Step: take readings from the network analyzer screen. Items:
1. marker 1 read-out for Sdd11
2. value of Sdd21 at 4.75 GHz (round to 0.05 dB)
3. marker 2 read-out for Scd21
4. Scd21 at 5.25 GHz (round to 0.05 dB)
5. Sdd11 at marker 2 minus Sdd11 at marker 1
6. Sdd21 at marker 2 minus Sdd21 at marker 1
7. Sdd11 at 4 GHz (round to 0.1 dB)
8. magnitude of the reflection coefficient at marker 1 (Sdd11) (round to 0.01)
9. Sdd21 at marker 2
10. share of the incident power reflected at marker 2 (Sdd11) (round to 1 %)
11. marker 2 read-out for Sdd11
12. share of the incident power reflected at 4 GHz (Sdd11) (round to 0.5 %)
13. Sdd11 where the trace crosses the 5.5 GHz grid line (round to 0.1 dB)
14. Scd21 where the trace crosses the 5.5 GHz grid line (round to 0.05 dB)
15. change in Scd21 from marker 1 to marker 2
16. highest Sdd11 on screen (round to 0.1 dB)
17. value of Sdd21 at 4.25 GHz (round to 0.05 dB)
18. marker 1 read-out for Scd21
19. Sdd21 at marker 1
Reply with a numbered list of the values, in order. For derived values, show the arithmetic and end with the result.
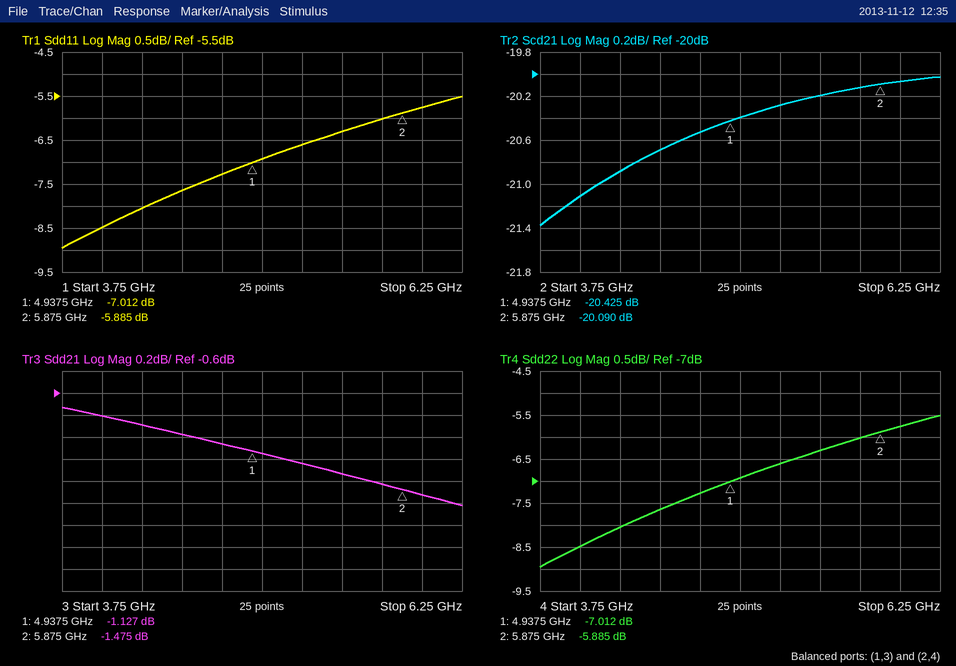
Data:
1. -7.012 dB
2. -1.05 dB
3. -20.090 dB
4. -20.30 dB
5. -5.885 − (-7.012) = 1.127 dB
6. -1.475 − (-1.127) = -0.348 dB
7. -8.5 dB
8. 10^(-7.012/20) ≈ 0.45
9. -1.475 dB
10. 10^(-5.885/10) ≈ 26 %
11. -5.885 dB
12. 10^(-8.5/10) ≈ 14.1 %, so 14.0 % to the nearest 0.5 %
13. -6.3 dB
14. -20.20 dB
15. -20.09 − (-20.425) = 0.335 dB
16. -5.5 dB
17. -0.90 dB
18. -20.425 dB
19. -1.127 dB
